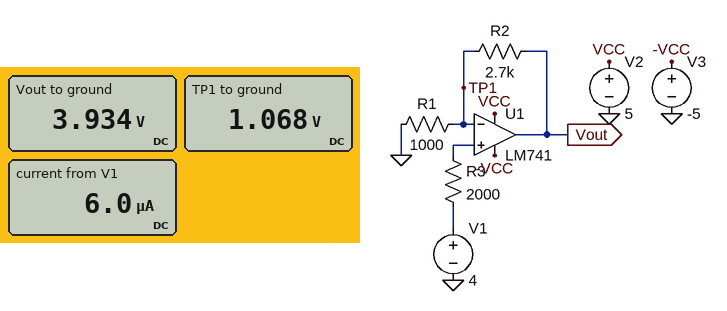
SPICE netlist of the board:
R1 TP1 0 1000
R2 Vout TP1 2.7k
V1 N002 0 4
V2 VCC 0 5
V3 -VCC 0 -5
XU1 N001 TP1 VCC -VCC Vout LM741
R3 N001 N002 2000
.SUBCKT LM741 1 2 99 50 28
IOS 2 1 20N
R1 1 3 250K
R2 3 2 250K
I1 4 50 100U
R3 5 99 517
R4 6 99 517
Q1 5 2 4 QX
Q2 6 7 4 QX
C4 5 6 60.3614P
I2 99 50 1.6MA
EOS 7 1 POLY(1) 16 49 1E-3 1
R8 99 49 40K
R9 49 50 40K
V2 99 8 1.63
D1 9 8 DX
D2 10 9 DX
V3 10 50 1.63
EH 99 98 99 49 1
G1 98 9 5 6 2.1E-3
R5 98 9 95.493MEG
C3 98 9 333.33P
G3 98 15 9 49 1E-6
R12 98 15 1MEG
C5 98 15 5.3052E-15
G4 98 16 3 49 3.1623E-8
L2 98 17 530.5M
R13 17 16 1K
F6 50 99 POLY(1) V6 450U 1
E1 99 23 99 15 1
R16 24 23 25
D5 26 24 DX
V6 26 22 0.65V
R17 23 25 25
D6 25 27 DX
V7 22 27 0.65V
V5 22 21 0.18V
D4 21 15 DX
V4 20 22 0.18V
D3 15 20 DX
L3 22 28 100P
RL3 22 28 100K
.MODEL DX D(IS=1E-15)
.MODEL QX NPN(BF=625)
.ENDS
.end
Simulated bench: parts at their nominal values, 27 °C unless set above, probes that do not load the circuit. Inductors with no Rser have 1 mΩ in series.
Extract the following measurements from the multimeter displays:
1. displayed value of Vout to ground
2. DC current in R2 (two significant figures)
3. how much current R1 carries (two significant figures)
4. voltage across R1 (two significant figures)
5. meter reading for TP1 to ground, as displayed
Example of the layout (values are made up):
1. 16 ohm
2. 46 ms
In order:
1. 3.934 V
2. 1.1 mA
3. 1.1 mA
4. 1.1 V
5. 1.068 V
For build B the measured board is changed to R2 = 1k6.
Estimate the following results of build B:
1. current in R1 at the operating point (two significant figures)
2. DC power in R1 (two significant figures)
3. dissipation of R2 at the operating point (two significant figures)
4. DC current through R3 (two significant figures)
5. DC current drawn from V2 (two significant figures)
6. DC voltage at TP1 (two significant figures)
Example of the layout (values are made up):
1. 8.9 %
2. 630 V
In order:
1. 1.5 mA
2. 2.3 mW
3. 3.6 mW
4. 5.1 µA
5. 2.9 mA
6. 1.5 V
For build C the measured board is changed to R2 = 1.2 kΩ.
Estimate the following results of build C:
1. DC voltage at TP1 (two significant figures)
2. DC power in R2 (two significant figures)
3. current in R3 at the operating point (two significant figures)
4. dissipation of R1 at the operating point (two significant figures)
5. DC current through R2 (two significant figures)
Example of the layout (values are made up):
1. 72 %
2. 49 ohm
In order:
1. 1.8 V
2. 3.8 mW
3. 4.6 µA
4. 3.2 mW
5. 1.8 mA
